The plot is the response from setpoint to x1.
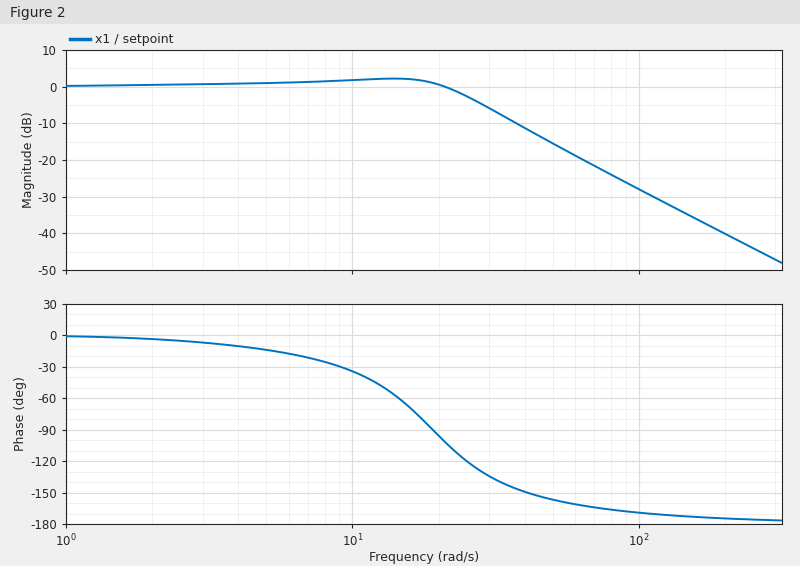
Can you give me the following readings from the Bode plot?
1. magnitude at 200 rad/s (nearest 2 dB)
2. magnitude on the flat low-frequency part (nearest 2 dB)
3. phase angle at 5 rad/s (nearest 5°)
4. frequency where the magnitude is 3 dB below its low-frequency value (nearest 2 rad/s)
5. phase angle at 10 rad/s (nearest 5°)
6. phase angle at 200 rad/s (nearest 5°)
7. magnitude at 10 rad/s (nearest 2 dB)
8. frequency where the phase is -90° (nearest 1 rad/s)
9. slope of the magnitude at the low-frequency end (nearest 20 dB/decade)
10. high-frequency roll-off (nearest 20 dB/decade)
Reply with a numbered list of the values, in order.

1. -40 dB
2. 0 dB
3. -15°
4. 26 rad/s
5. -35°
6. -175°
7. 2 dB
8. 19 rad/s
9. 0 dB/decade
10. -40 dB/decade
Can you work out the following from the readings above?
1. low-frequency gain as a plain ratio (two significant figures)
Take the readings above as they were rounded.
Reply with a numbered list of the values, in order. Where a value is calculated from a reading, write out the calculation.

1. 10^(0 / 20) = 1.0
